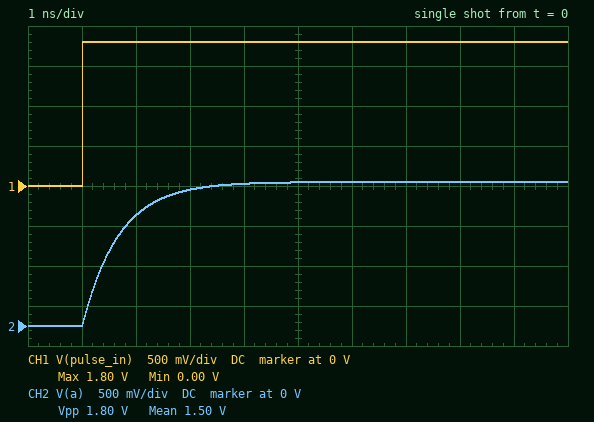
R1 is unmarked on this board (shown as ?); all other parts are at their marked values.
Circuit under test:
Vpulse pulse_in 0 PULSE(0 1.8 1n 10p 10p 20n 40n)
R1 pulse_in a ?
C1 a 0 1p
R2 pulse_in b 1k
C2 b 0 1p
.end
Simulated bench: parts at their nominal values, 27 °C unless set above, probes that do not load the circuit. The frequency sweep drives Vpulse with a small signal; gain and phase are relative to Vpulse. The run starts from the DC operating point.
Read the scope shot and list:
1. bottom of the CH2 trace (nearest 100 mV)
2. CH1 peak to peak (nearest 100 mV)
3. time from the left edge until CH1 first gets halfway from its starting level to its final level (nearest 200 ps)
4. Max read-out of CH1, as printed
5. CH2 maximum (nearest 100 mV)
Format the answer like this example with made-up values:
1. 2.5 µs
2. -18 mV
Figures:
1. 0 V
2. 1.8 V
3. 1.0 ns
4. 1.80 V
5. 1.8 V
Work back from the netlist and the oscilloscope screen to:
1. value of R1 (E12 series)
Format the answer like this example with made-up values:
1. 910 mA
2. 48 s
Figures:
1. 680 Ω
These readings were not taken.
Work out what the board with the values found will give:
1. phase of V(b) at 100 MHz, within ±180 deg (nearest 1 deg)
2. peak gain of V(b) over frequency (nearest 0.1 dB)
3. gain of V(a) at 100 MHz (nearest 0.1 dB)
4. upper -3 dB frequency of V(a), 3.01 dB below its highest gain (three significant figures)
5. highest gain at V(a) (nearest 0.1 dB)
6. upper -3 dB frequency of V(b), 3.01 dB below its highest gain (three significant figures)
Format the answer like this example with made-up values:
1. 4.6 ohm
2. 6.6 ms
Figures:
1. -32 deg
2. 0 dB
3. -0.7 dB
4. 234 MHz
5. 0 dB
6. 159 MHz
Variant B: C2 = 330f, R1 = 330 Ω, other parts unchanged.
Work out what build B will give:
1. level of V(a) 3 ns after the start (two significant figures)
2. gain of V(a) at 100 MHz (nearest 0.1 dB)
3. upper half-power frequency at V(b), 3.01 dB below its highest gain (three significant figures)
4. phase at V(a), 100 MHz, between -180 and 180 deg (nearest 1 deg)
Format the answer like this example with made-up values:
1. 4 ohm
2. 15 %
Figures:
1. 1.8 V
2. -0.2 dB
3. 482 MHz
4. -12 deg
